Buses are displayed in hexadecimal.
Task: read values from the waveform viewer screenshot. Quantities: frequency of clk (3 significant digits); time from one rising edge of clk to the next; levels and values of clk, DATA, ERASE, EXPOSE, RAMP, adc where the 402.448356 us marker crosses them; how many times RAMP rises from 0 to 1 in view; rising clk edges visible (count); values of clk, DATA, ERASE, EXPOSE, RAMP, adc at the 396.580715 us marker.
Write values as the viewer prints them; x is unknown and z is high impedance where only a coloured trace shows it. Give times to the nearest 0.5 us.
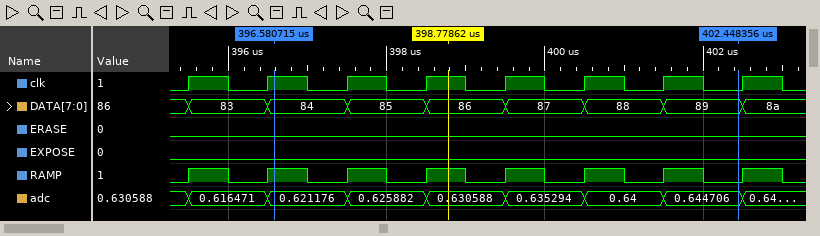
1.00 MHz
1 us
clk=0, DATA=89, ERASE=0, EXPOSE=0, RAMP=0, adc=0.644706
8
8
clk=1, DATA=84, ERASE=0, EXPOSE=0, RAMP=1, adc=0.621176
